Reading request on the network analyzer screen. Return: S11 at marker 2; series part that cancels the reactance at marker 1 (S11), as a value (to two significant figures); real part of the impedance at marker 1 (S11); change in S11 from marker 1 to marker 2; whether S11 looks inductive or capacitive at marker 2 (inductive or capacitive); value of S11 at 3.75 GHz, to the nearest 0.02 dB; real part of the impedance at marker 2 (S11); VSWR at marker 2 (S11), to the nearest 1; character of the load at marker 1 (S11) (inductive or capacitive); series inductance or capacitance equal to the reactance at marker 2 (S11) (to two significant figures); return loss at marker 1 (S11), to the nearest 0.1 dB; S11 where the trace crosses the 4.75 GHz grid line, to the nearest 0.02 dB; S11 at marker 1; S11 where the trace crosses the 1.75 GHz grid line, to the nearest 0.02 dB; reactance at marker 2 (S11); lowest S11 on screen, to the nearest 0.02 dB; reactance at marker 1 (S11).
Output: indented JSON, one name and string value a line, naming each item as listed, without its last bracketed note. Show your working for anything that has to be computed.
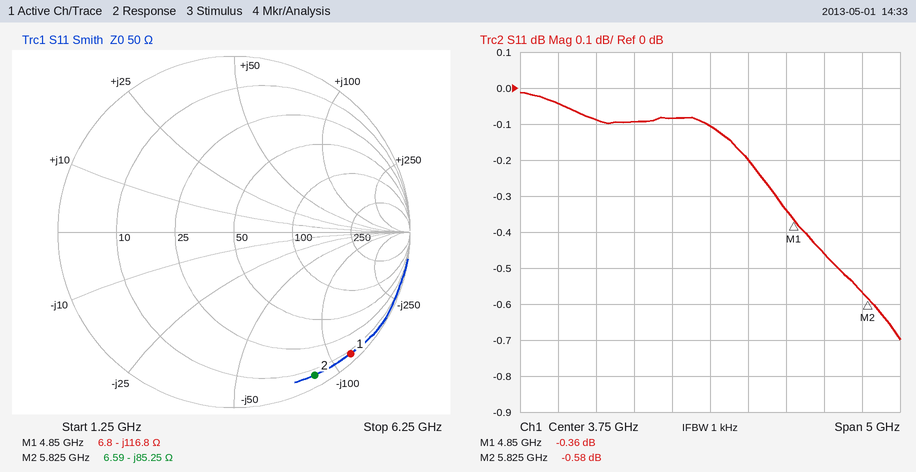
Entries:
{
  "S11 at marker 2": "-0.58 dB",
  "series part that cancels the reactance at marker 1 (S11), as a value": "L = 116.8 Ω/(2π × 4.85 GHz) ≈ 3.8 nH",
  "real part of the impedance at marker 1": "6.8 Ω",
  "change in S11 from marker 1 to marker 2": "-0.58 − (-0.36) = -0.22 dB",
  "whether S11 looks inductive or capacitive at marker 2": "capacitive",
  "value of S11 at 3.75 GHz, to the nearest 0.02 dB": "-0.10 dB",
  "real part of the impedance at marker 2": "6.59 Ω",
  "VSWR at marker 2 (S11), to the nearest 1": "(1 + 0.9354)/(1 − 0.9354) ≈ 30",
  "character of the load at marker 1 (S11)": "capacitive",
  "series inductance or capacitance equal to the reactance at marker 2 (S11)": "C = 1/(2π × 5.825 GHz × 85.25 Ω) ≈ 321 fF, so 320 fF to two significant figures",
  "return loss at marker 1 (S11), to the nearest 0.1 dB": "0.4 dB",
  "S11 where the trace crosses the 4.75 GHz grid line, to the nearest 0.02 dB": "-0.34 dB",
  "S11 at marker 1": "-0.36 dB",
  "S11 where the trace crosses the 1.75 GHz grid line, to the nearest 0.02 dB": "-0.04 dB",
  "reactance at marker 2": "-85.25 Ω",
  "lowest S11 on screen, to the nearest 0.02 dB": "-0.70 dB",
  "reactance at marker 1": "-116.8 Ω"
}
